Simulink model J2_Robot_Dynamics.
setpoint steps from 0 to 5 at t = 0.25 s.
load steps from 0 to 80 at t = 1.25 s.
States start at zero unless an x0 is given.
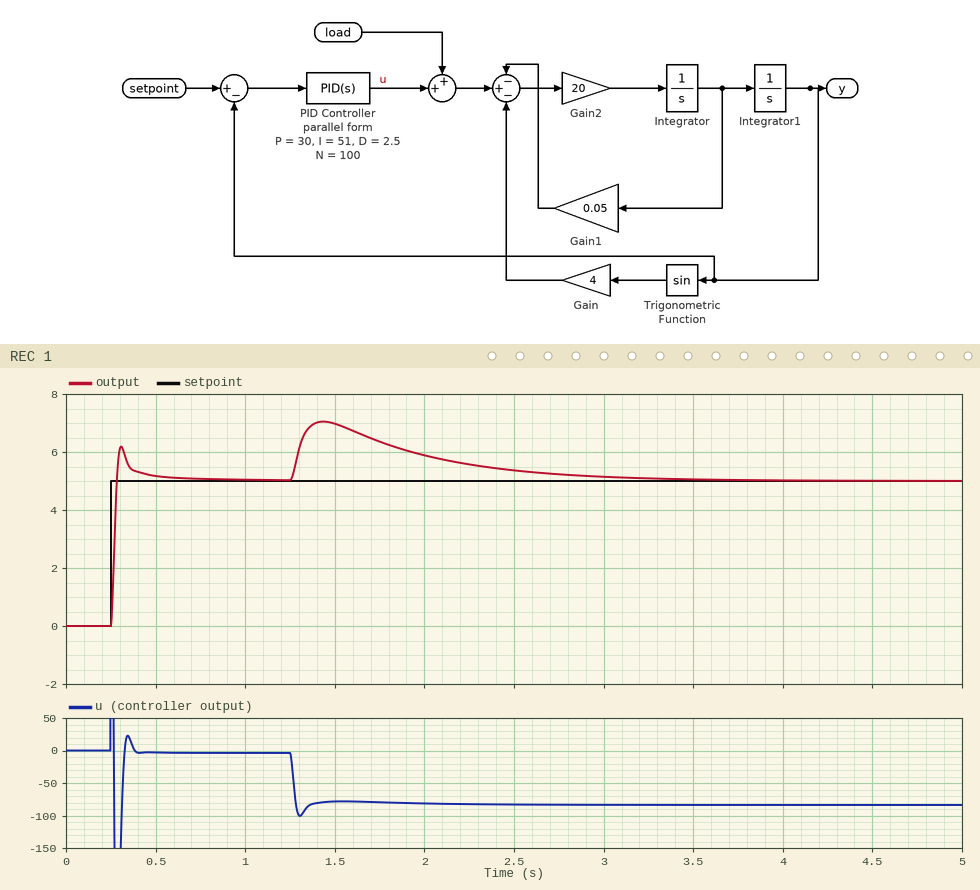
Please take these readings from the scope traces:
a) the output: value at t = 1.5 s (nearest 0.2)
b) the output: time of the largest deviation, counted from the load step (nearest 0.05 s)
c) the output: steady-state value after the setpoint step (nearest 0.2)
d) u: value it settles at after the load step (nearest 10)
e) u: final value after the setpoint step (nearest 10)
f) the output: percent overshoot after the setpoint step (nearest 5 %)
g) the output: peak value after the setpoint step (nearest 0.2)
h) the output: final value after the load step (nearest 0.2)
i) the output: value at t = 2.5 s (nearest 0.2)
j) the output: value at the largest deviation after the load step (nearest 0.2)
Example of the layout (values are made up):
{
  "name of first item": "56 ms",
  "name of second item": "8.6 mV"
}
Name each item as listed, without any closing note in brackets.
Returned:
{
  "the output: value at t = 1.5 s": "7.0",
  "the output: time of the largest deviation, counted from the load step": "0.20 s",
  "the output: steady-state value after the setpoint step": "5.0",
  "u: value it settles at after the load step": "-80",
  "u: final value after the setpoint step": "0",
  "the output: percent overshoot after the setpoint step": "25 %",
  "the output: peak value after the setpoint step": "6.2",
  "the output: final value after the load step": "5.0",
  "the output: value at t = 2.5 s": "5.4",
  "the output: value at the largest deviation after the load step": "7.0"
}
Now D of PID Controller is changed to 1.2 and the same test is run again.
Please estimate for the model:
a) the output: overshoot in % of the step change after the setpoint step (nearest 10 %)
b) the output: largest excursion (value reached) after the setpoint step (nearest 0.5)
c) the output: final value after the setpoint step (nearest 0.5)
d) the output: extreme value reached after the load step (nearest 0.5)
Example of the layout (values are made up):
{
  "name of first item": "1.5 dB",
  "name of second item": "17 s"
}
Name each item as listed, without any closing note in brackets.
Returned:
{
  "the output: overshoot in % of the step change after the setpoint step": "40 %",
  "the output: largest excursion (value reached) after the setpoint step": "7.0",
  "the output: final value after the setpoint step": "5.0",
  "the output: extreme value reached after the load step": "7.5"
}
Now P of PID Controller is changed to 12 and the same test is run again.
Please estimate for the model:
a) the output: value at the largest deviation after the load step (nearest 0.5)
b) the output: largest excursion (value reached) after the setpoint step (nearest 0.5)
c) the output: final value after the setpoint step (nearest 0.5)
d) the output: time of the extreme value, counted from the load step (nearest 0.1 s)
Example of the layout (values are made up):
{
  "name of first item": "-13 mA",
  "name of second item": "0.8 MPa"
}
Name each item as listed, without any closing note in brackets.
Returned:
{
  "the output: value at the largest deviation after the load step": "8.5",
  "the output: largest excursion (value reached) after the setpoint step": "5.5",
  "the output: final value after the setpoint step": "5.0",
  "the output: time of the extreme value, counted from the load step": "0.3 s"
}
